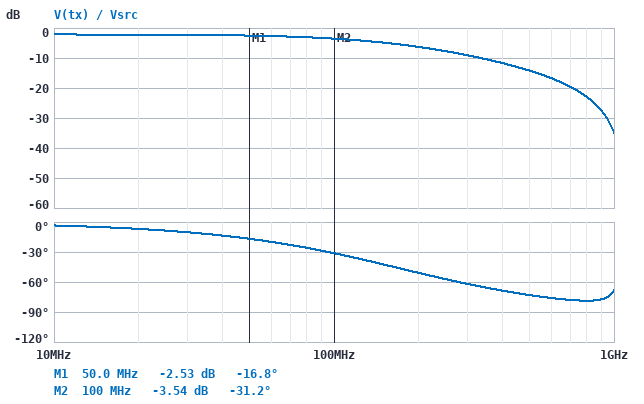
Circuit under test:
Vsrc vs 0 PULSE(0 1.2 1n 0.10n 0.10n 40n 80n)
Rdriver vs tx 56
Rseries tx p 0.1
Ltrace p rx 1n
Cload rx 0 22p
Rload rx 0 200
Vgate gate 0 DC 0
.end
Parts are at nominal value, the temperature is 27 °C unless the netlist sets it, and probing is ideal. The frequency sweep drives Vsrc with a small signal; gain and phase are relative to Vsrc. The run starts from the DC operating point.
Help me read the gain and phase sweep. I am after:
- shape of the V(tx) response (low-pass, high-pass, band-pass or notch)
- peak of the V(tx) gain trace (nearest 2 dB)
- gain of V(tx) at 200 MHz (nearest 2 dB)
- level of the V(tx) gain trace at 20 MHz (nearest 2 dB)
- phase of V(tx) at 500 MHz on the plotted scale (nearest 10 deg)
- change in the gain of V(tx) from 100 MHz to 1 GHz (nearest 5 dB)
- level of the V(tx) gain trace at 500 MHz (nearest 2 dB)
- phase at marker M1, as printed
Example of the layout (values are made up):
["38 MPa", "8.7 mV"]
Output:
["low-pass", "-2 dB", "-6 dB", "-2 dB", "-70 deg", "-30 dB", "-14 dB", "-16.8 deg"]
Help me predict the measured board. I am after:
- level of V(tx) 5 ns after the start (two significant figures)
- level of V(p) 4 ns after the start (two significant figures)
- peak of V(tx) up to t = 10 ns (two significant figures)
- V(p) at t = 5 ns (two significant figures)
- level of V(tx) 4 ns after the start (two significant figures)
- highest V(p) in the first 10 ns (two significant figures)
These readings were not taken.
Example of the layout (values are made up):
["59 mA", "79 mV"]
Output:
["920 mV", "890 mV", "940 mV", "920 mV", "890 mV", "940 mV"]
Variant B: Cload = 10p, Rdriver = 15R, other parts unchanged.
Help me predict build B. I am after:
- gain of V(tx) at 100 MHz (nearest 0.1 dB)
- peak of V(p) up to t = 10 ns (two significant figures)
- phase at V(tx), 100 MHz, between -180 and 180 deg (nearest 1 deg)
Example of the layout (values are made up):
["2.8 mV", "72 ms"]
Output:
["-0.7 dB", "1.1 V", "-5 deg"]
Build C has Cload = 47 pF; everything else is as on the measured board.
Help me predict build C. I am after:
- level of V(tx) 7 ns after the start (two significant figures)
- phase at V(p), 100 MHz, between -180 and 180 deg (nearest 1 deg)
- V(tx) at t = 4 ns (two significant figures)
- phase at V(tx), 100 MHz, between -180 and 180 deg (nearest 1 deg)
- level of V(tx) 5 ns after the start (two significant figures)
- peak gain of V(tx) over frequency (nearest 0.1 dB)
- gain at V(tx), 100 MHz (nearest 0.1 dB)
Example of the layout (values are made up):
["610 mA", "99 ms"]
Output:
["890 mV", "-53 deg", "710 mV", "-52 deg", "800 mV", "-2.1 dB", "-6.5 dB"]
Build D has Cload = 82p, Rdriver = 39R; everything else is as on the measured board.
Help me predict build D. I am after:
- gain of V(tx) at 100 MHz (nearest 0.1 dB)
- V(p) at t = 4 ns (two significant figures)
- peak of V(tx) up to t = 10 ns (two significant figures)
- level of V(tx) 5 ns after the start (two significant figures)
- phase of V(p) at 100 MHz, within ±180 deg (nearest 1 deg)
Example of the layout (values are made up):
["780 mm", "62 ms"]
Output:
["-7.6 dB", "670 mV", "970 mV", "770 mV", "-60 deg"]
